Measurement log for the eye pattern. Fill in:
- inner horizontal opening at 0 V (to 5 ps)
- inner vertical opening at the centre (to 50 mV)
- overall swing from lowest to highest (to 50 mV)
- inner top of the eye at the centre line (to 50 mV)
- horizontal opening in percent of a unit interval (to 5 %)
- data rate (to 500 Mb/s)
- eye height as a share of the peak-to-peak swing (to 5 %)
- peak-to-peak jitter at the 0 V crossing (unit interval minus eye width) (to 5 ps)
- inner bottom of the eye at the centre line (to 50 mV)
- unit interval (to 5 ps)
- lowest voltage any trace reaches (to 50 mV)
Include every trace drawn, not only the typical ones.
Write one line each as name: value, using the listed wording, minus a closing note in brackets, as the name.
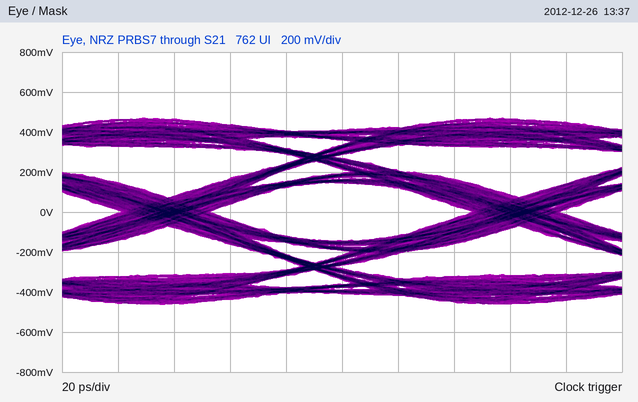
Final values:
inner horizontal opening at 0 V: 95 ps
inner vertical opening at the centre: 300 mV
overall swing from lowest to highest: 950 mV
inner top of the eye at the centre line: 150 mV
horizontal opening in percent of a unit interval: 75 %
data rate: 8.0 Gb/s
eye height as a share of the peak-to-peak swing: 30 %
peak-to-peak jitter at the 0 V crossing (unit interval minus eye width): 30 ps
inner bottom of the eye at the centre line: -150 mV
unit interval: 125 ps
lowest voltage any trace reaches: -450 mV
